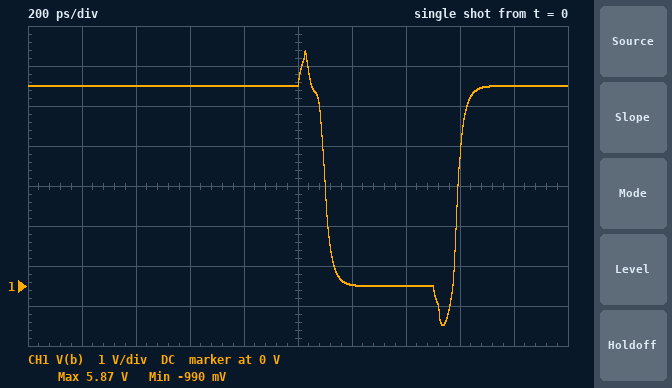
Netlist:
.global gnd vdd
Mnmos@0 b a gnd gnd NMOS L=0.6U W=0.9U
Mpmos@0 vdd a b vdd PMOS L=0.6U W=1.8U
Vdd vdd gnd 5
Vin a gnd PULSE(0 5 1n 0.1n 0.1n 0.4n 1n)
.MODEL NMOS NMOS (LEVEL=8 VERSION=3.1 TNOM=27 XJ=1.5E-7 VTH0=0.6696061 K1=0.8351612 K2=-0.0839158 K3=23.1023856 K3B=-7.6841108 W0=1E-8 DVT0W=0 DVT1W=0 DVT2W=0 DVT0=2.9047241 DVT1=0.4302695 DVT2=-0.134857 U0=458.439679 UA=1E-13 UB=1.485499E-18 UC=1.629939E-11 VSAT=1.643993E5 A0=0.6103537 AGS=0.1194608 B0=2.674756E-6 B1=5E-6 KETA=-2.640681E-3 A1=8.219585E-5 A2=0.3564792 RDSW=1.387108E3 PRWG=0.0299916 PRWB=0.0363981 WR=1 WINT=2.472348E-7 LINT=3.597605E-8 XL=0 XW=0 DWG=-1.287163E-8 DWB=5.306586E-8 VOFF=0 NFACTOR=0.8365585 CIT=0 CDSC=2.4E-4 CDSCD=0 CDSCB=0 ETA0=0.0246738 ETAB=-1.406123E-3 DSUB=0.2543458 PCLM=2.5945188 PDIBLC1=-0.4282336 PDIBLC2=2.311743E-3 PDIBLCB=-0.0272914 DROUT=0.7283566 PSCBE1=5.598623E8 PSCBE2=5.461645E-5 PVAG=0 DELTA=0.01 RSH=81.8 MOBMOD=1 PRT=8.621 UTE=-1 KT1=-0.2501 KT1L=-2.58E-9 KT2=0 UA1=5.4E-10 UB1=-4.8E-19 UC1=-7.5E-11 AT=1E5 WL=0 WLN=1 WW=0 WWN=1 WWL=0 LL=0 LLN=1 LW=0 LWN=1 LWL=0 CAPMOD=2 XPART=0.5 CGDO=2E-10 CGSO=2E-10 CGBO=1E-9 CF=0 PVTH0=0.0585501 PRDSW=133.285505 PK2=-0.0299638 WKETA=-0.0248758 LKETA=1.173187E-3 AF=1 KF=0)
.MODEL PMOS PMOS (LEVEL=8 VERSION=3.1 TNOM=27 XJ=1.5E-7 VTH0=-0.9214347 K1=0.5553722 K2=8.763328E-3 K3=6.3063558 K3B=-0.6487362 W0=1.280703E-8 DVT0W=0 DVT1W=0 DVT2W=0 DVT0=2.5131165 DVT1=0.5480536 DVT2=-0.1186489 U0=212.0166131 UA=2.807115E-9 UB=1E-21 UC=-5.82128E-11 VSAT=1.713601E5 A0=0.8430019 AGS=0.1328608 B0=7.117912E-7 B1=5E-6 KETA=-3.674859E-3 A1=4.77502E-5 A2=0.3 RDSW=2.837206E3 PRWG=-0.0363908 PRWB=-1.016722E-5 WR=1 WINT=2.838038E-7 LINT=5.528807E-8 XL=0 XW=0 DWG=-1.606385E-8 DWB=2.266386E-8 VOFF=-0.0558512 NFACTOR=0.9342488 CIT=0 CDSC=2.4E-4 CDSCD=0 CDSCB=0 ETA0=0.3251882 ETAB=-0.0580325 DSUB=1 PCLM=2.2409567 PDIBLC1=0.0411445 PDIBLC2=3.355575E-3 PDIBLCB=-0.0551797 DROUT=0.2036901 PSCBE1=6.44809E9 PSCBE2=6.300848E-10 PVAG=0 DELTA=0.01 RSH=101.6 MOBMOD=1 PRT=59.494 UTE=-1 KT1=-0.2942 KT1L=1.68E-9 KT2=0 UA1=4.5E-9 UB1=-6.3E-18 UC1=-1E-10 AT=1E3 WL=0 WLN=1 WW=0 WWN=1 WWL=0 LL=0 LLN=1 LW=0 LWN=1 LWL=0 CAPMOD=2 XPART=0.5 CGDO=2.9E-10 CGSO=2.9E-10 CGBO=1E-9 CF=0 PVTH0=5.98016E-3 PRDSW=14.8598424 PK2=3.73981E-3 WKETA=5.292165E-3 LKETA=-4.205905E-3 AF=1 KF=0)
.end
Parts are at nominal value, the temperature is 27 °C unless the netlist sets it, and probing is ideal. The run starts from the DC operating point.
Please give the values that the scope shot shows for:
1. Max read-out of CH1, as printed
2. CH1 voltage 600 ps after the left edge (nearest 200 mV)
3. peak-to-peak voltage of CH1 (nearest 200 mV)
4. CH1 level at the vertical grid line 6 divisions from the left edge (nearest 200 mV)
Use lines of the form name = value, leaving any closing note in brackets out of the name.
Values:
Max read-out of CH1, as printed = 5.87 V
CH1 voltage 600 ps after the left edge = 5.0 V
peak-to-peak voltage of CH1 = 6.8 V
CH1 level at the vertical grid line 6 divisions from the left edge = 0 V
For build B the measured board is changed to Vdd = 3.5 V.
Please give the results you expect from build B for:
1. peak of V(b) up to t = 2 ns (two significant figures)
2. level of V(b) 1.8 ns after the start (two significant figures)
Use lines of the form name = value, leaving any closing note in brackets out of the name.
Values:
peak of V(b) up to t = 2 ns = 4.3 V
level of V(b) 1.8 ns after the start = 3.5 V
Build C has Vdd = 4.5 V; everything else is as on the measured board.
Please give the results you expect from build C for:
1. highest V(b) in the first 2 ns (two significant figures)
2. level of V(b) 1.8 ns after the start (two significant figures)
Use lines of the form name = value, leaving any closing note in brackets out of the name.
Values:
highest V(b) in the first 2 ns = 5.4 V
level of V(b) 1.8 ns after the start = 4.5 V
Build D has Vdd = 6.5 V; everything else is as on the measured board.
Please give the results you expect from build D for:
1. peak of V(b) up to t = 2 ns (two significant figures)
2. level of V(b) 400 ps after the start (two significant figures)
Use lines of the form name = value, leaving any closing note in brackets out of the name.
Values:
peak of V(b) up to t = 2 ns = 7.4 V
level of V(b) 400 ps after the start = 6.5 V
